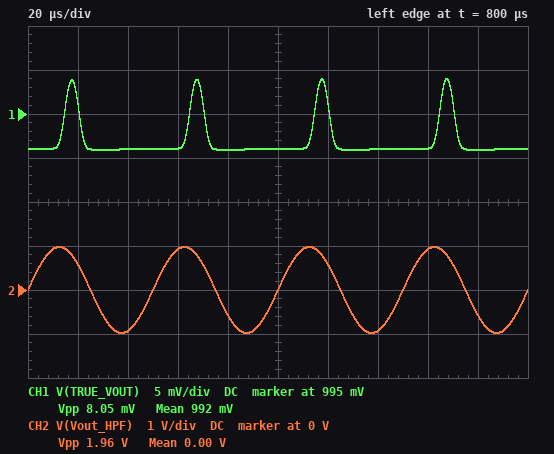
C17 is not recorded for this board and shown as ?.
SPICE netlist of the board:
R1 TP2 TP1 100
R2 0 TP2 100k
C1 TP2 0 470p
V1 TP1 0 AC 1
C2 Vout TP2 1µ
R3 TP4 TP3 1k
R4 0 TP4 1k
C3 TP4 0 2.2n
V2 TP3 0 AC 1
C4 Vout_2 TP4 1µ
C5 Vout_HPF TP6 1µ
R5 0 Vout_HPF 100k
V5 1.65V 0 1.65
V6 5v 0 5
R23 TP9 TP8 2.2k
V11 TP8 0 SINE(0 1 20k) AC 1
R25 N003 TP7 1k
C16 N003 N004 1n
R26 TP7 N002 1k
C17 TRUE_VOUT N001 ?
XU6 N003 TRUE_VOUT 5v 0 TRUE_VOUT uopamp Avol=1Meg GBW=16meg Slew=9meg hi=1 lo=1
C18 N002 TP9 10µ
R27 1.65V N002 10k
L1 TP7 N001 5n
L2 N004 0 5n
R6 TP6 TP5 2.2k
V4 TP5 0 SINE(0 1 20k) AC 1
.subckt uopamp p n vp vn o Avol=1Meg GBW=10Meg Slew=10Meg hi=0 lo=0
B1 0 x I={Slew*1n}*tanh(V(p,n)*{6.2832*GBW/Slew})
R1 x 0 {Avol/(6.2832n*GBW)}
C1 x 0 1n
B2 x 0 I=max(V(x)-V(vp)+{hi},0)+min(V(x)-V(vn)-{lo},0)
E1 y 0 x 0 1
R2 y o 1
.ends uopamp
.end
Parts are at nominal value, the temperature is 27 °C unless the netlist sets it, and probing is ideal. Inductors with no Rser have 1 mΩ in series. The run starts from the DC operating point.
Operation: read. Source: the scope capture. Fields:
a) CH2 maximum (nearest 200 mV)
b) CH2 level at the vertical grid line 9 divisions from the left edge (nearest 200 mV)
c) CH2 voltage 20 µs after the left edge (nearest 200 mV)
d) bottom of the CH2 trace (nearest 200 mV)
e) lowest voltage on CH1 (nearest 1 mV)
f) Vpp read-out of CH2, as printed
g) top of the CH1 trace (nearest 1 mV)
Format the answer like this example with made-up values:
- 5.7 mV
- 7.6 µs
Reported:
- 1.0 V
- -600 mV
- 600 mV
- -1.0 V
- 991 mV
- 1.96 V
- 999 mV
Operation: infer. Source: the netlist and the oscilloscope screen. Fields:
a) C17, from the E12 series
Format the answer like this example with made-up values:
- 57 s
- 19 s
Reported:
- 680 pF
